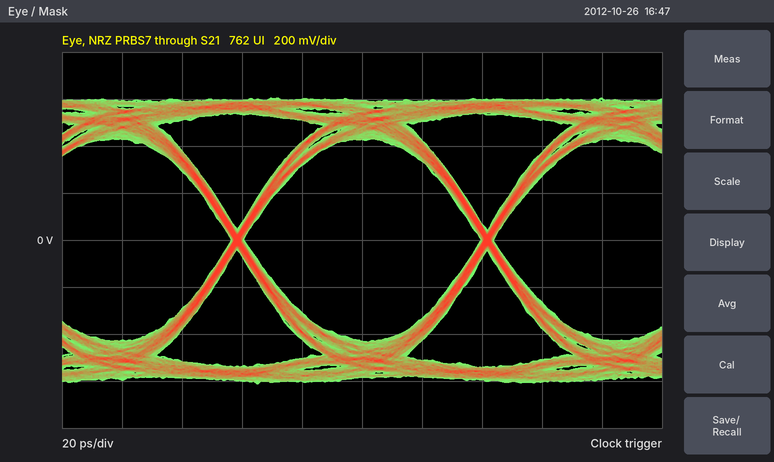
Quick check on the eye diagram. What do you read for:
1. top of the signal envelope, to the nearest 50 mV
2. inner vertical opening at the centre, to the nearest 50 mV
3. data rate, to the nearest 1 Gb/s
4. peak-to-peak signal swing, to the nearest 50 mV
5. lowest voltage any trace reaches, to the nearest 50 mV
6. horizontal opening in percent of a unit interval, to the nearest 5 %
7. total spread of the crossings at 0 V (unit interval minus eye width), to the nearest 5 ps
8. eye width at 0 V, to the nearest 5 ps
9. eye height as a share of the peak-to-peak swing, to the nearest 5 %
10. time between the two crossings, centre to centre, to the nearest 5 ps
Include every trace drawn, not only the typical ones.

600 mV
850 mV
12 Gb/s
1.20 V
-600 mV
95 %
5 ps
80 ps
70 %
85 ps
